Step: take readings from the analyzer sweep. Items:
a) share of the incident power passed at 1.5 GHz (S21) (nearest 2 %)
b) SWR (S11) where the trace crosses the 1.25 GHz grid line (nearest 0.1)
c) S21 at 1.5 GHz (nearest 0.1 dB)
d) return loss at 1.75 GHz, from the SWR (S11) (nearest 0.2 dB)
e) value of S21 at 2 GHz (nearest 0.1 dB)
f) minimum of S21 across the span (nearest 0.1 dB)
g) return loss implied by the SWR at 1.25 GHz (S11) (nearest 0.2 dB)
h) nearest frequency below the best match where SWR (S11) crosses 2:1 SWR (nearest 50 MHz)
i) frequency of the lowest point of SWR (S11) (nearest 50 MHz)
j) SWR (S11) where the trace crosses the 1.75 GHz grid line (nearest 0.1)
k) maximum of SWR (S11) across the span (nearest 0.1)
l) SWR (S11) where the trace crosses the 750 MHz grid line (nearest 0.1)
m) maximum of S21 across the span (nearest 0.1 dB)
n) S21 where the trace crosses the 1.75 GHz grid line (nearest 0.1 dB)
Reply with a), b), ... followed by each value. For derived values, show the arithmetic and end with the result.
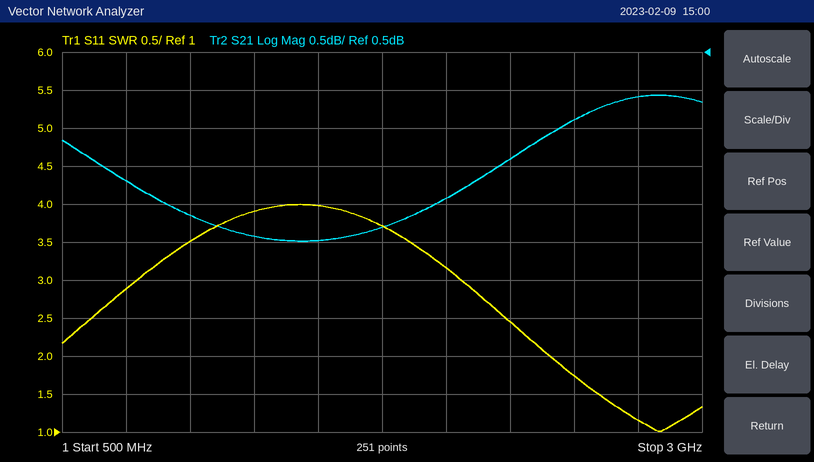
a) 10^(-2/10) ≈ 63.1 %, so 64 % to the nearest 2 %
b) 3.9
c) -2.0 dB
d) −20 log10((3.7 − 1)/(3.7 + 1)) ≈ 4.8 dB
e) -1.4 dB
f) -2.0 dB
g) −20 log10((3.9 − 1)/(3.9 + 1)) ≈ 4.6 dB
h) 2.40 GHz
i) 2.85 GHz
j) 3.7
k) 4.0
l) 2.9
m) -0.1 dB
n) -1.8 dB
